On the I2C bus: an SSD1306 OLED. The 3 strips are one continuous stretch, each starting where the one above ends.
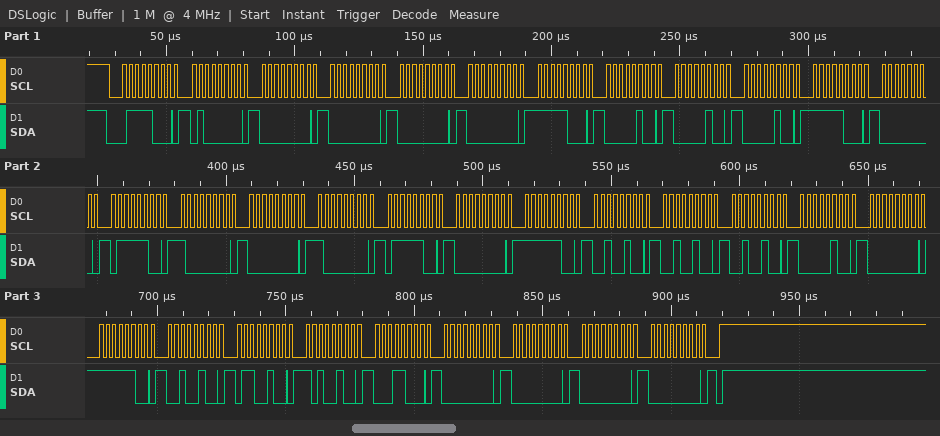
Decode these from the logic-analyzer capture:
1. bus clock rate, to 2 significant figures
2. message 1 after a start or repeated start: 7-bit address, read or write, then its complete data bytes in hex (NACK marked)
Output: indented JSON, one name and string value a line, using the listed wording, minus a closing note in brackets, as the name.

{
  "bus clock rate, to 2 significant figures": "400 kHz",
  "message 1 after a start or repeated start: 7-bit address, read or write, then its complete data bytes in hex": "0x3C write: 40 00 00 00 00 F8 04 04 04 F8 00 7C 80 00 80 7C 00 FC 24 24 24 04 00 FC 24 64 A4 18 00 00 00 00"
}
